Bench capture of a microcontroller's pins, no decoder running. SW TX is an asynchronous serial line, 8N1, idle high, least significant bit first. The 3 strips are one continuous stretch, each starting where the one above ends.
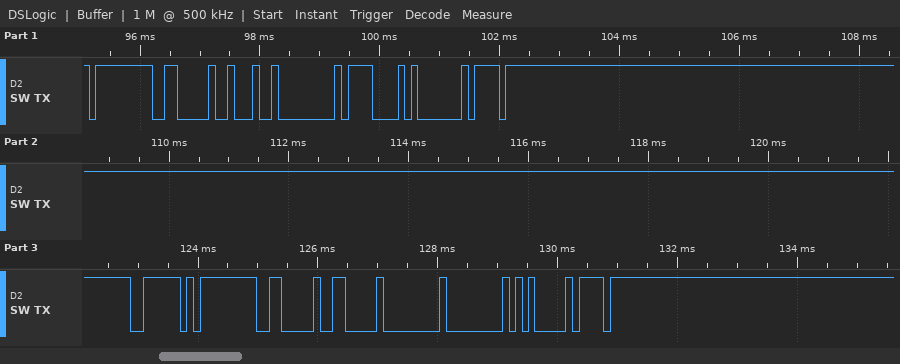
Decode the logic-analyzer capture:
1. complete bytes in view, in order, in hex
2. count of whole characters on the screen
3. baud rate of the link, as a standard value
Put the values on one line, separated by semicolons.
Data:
0xFF 0x06 0x22 0x00 0x0F 0x01 0xEF 0x7E 0xFF 0x06 0x06 0x00 0x00 0x05 0xEF; 15; 9600 baud
